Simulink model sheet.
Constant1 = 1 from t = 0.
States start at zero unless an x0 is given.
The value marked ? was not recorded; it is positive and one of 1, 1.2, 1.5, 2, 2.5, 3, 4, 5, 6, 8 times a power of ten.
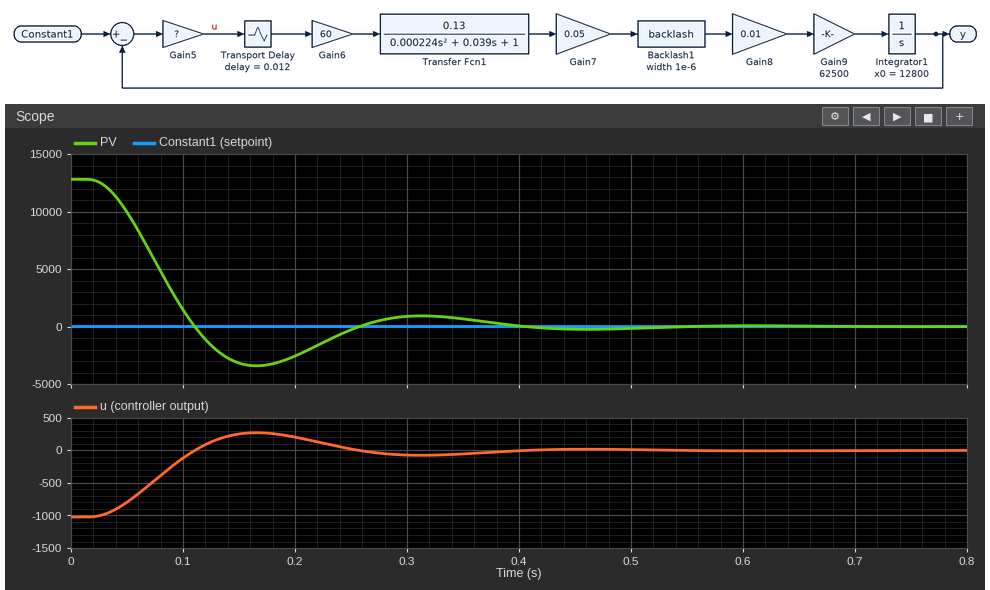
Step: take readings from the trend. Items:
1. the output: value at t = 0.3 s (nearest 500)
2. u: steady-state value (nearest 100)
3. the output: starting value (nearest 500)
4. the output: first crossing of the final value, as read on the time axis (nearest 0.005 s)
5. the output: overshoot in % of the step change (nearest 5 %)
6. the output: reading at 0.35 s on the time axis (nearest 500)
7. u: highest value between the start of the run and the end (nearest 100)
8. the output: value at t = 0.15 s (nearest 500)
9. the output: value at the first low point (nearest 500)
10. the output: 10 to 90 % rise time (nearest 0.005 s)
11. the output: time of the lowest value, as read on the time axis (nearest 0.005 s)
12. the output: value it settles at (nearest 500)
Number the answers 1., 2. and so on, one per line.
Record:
1. 1000
2. 0
3. 13000
4. 0.110 s
5. 25 %
6. 500
7. 300
8. -3000
9. -3500
10. 0.065 s
11. 0.165 s
12. 0
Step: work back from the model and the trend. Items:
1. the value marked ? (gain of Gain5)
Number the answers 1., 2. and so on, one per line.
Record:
1. 0.08
